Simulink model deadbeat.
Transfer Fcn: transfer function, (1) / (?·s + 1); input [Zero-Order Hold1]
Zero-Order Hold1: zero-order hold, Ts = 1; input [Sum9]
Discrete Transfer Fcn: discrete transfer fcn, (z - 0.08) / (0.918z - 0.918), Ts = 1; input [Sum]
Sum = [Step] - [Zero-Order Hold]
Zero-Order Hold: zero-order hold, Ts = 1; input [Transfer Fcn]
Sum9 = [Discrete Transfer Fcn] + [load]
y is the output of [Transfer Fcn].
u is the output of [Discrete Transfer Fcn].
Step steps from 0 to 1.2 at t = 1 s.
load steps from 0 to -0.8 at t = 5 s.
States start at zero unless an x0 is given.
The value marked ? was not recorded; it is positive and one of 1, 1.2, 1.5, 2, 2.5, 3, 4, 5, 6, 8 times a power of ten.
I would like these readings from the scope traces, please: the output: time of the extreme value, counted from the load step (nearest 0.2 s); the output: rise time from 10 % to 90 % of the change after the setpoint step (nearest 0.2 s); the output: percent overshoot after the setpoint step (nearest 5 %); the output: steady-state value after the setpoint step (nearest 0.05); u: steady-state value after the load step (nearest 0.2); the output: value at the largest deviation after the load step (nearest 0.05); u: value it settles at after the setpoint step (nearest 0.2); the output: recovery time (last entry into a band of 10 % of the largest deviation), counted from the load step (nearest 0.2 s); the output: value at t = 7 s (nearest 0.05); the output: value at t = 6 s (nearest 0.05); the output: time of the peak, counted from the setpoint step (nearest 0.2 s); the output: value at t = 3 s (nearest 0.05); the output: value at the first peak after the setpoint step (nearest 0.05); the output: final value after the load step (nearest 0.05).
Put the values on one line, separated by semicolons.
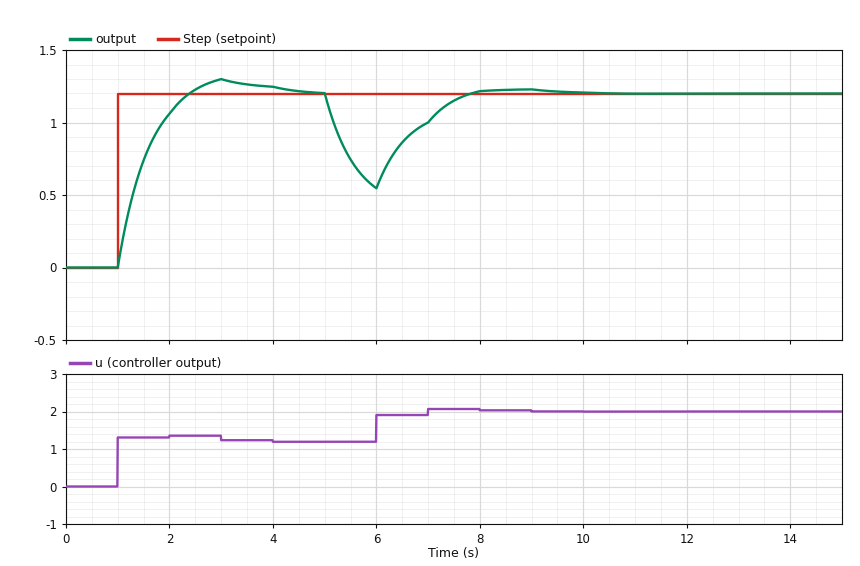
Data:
1.0 s; 1.0 s; 10 %; 1.20; 2.0; 0.55; 1.2; 2.4 s; 1.00; 0.55; 2.0 s; 1.30; 1.30; 1.20
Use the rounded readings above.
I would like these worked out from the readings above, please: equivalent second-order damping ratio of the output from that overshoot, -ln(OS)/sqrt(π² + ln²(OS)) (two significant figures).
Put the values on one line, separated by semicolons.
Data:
0.59
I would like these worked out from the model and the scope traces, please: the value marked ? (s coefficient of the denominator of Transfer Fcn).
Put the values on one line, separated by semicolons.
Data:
0.6
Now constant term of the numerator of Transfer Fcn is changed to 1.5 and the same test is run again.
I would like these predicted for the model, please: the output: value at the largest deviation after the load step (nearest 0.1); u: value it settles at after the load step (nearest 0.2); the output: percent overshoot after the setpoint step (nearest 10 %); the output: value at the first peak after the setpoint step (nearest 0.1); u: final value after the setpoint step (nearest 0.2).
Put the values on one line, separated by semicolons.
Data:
0.2; 1.6; 30 %; 1.6; 0.8
